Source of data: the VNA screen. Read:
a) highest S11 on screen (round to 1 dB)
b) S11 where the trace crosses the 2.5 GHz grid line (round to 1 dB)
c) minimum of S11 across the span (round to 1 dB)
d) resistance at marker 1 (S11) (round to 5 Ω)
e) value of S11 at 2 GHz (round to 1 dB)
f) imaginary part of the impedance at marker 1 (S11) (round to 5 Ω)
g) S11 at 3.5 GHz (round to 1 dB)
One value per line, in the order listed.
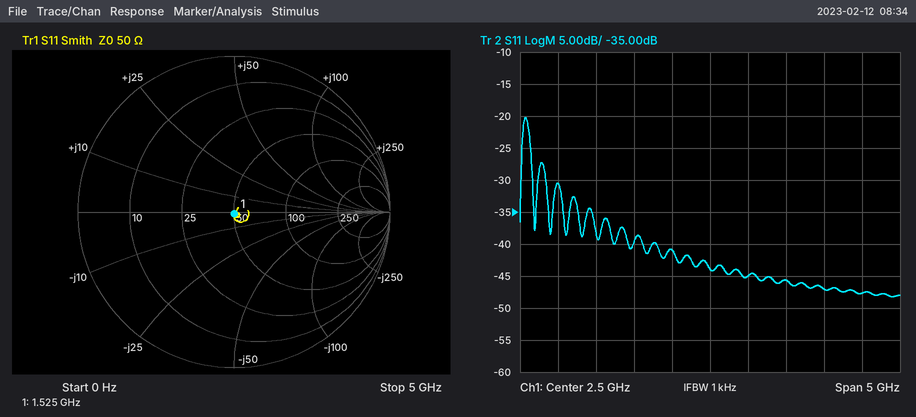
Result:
-20 dB
-44 dB
-48 dB
50 Ω
-41 dB
0 Ω
-46 dB
